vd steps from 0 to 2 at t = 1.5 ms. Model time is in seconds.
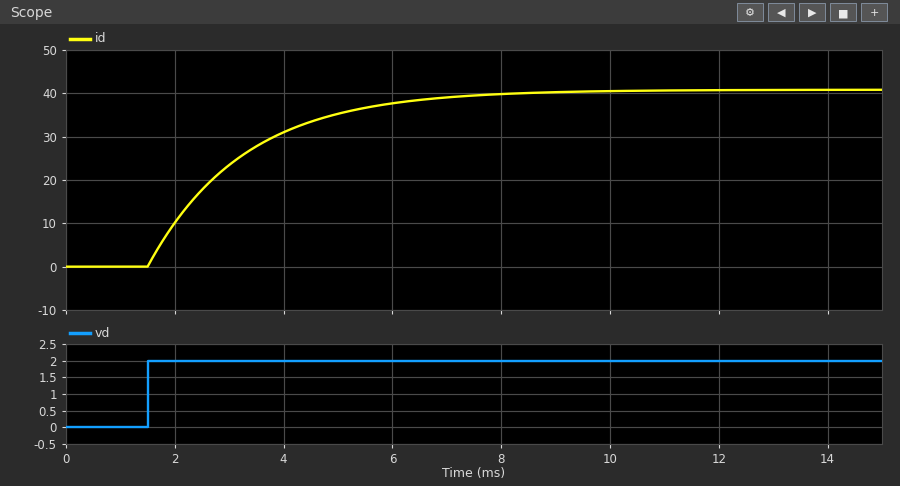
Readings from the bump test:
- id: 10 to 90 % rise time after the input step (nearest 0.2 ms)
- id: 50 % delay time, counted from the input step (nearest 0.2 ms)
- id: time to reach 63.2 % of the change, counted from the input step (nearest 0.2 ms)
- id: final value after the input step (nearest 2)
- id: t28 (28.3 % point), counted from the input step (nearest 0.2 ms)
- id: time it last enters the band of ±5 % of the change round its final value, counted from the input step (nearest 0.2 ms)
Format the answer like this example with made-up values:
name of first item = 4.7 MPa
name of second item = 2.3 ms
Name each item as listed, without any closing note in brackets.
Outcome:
id: 10 to 90 % rise time after the input step = 3.8 ms
id: 50 % delay time, counted from the input step = 1.2 ms
id: time to reach 63.2 % of the change, counted from the input step = 1.8 ms
id: final value after the input step = 40
id: t28 (28.3 % point), counted from the input step = 0.6 ms
id: time it last enters the band of ±5 % of the change round its final value, counted from the input step = 5.2 ms
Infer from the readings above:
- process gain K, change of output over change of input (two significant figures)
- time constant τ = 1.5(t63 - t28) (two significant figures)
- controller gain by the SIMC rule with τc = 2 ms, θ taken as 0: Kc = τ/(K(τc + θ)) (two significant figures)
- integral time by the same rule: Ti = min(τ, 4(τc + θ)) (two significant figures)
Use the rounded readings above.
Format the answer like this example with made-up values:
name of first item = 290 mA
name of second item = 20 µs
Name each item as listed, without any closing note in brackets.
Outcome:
process gain K, change of output over change of input = 20
time constant τ = 1.5(t63 - t28) = 1.8 ms
controller gain by the SIMC rule with τc = 2 ms, θ taken as 0: Kc = τ/(K(τc + θ)) = 0.045
integral time by the same rule: Ti = min(τ, 4(τc + θ)) = 1.8 ms
